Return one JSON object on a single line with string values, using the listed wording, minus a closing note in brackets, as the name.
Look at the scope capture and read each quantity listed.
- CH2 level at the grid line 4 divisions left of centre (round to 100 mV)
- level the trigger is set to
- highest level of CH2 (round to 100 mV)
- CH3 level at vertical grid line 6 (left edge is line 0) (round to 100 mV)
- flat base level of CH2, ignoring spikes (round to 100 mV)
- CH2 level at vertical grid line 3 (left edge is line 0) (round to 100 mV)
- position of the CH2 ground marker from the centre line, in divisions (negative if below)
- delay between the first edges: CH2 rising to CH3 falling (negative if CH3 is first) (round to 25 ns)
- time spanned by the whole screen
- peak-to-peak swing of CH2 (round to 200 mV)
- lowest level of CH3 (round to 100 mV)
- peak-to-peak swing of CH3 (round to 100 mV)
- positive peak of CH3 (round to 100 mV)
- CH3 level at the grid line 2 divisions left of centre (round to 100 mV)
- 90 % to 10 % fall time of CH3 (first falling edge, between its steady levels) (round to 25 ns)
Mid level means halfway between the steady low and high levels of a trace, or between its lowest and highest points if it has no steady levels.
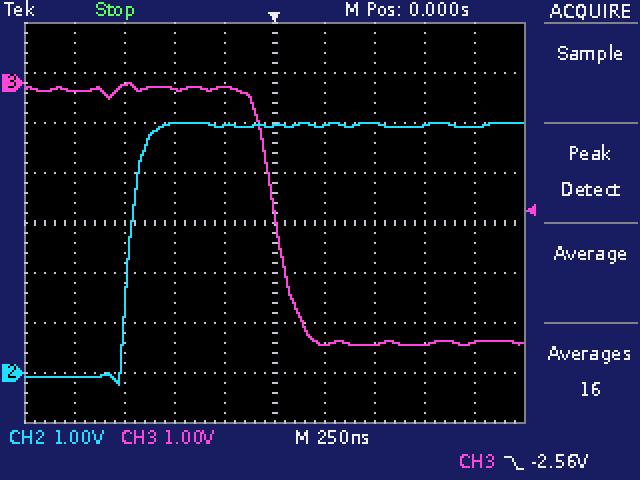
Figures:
{"CH2 level at the grid line 4 divisions left of centre": "-100 mV", "level the trigger is set to": "-2.56 V", "highest level of CH2": "5.0 V", "CH3 level at vertical grid line 6 (left edge is line 0)": "-5.2 V", "flat base level of CH2, ignoring spikes": "-100 mV", "CH2 level at vertical grid line 3 (left edge is line 0)": "5.0 V", "position of the CH2 ground marker from the centre line, in divisions": "-3.0 div", "delay between the first edges: CH2 rising to CH3 falling (negative if CH3 is first)": "+725 ns", "time spanned by the whole screen": "2.5 µs", "peak-to-peak swing of CH2": "5.2 V", "lowest level of CH3": "-5.2 V", "peak-to-peak swing of CH3": "5.2 V", "positive peak of CH3": "0.0 V", "CH3 level at the grid line 2 divisions left of centre": "-100 mV", "90 % to 10 % fall time of CH3 (first falling edge, between its steady levels)": "225 ns"}
